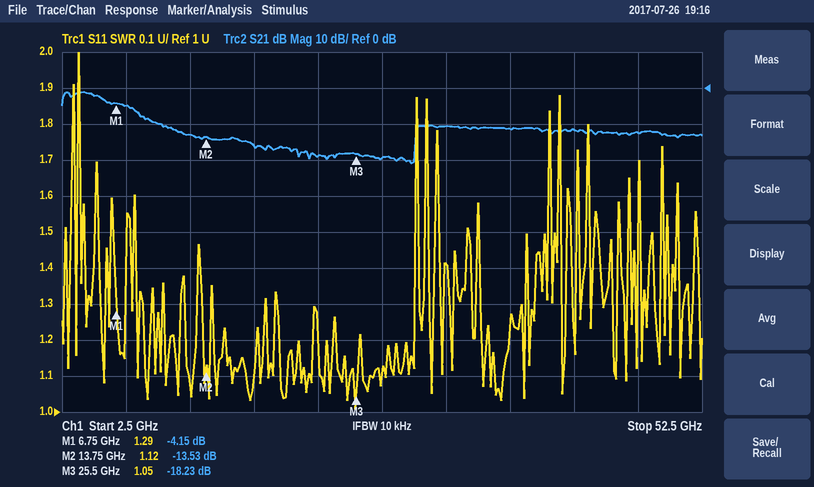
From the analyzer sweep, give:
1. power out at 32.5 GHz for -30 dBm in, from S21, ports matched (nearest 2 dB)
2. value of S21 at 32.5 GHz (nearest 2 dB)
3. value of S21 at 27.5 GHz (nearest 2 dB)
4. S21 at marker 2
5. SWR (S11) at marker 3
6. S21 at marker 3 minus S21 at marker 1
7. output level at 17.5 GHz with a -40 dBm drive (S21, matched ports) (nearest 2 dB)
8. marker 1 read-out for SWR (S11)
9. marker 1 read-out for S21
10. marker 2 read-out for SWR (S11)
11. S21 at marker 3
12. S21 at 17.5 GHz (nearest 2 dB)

-40 dBm
-10 dB
-20 dB
-13.53 dB
1.05
-14.08 dB
-56 dBm
1.29
-4.15 dB
1.12
-18.23 dB
-16 dB
